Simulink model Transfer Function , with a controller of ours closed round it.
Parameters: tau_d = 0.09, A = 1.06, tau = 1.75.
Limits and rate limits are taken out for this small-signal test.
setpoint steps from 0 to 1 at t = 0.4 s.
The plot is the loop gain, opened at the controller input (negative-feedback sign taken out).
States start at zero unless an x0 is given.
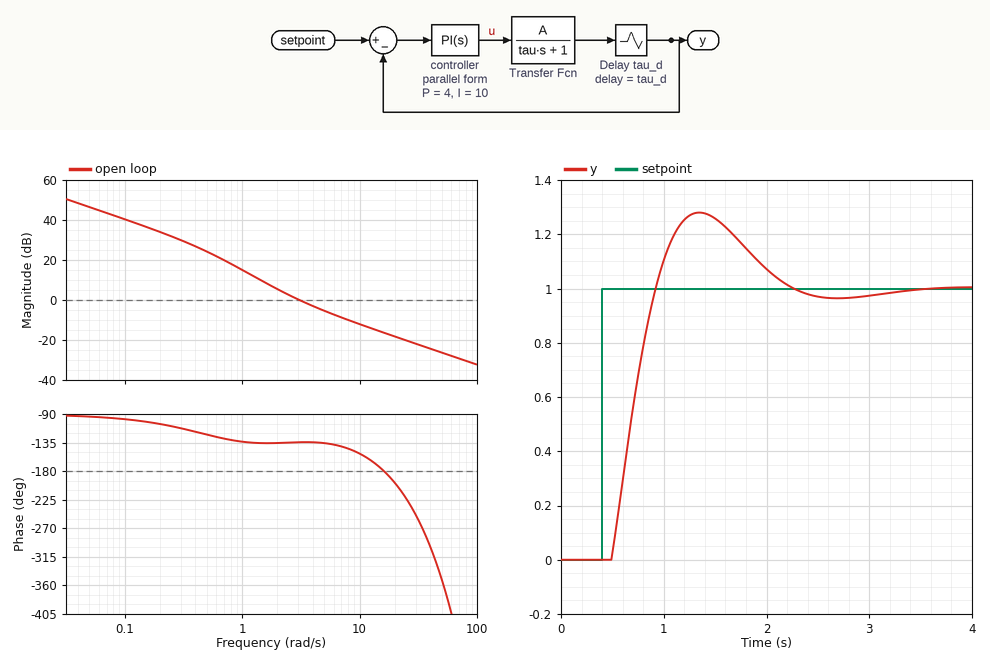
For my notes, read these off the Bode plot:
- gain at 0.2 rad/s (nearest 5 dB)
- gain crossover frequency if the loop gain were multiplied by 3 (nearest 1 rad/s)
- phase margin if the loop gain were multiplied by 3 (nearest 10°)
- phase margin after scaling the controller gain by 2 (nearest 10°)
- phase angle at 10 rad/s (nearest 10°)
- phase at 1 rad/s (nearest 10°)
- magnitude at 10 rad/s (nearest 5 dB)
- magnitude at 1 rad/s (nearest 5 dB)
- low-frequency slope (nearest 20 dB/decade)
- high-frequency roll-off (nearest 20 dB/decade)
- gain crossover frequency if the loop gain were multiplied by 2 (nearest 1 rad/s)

35 dB
8 rad/s
40°
40°
-150°
-130°
-10 dB
15 dB
-20 dB/decade
-20 dB/decade
5 rad/s
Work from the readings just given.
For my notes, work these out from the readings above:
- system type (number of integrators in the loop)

1
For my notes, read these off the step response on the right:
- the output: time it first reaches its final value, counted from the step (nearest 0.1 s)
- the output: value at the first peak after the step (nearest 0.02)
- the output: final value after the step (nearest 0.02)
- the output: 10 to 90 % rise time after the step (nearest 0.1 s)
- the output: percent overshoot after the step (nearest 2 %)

0.5 s
1.28
1.00
0.3 s
28 %
